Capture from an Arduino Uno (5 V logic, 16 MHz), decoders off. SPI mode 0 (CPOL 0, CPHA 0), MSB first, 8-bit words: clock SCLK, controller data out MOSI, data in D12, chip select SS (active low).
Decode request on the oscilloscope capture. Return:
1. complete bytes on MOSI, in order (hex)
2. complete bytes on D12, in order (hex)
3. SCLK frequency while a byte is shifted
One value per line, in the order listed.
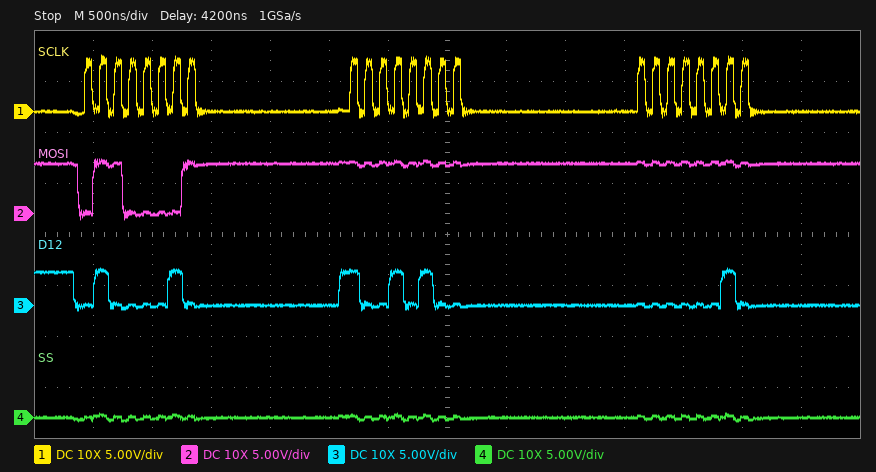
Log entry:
61 FF FF
42 94 02
8 MHz
